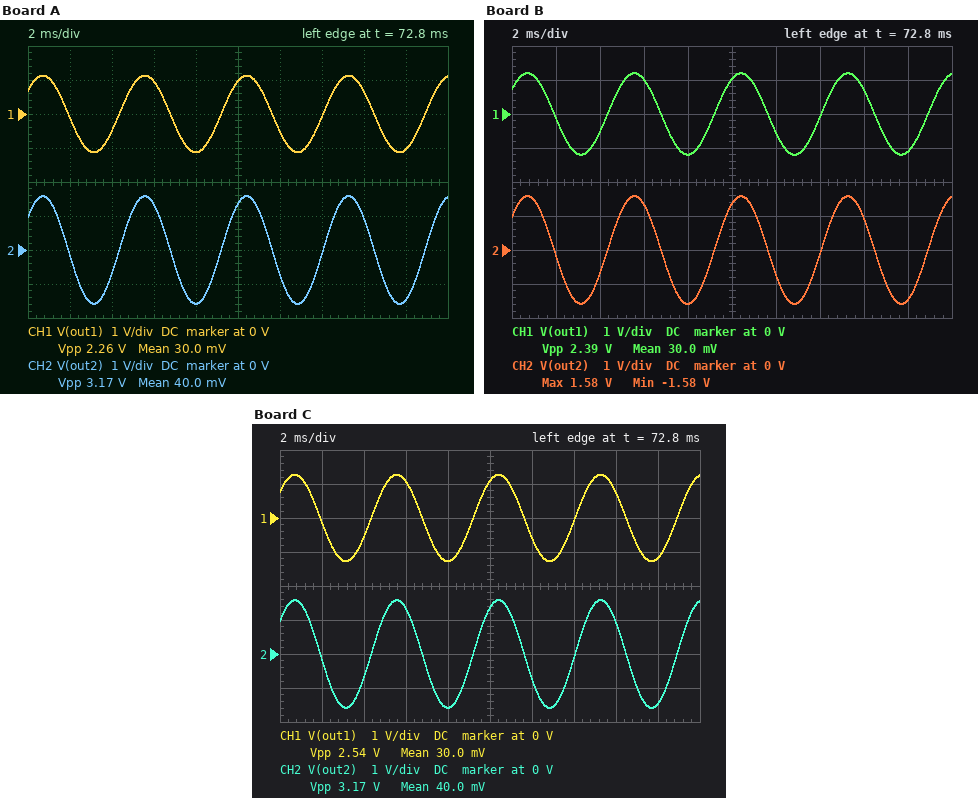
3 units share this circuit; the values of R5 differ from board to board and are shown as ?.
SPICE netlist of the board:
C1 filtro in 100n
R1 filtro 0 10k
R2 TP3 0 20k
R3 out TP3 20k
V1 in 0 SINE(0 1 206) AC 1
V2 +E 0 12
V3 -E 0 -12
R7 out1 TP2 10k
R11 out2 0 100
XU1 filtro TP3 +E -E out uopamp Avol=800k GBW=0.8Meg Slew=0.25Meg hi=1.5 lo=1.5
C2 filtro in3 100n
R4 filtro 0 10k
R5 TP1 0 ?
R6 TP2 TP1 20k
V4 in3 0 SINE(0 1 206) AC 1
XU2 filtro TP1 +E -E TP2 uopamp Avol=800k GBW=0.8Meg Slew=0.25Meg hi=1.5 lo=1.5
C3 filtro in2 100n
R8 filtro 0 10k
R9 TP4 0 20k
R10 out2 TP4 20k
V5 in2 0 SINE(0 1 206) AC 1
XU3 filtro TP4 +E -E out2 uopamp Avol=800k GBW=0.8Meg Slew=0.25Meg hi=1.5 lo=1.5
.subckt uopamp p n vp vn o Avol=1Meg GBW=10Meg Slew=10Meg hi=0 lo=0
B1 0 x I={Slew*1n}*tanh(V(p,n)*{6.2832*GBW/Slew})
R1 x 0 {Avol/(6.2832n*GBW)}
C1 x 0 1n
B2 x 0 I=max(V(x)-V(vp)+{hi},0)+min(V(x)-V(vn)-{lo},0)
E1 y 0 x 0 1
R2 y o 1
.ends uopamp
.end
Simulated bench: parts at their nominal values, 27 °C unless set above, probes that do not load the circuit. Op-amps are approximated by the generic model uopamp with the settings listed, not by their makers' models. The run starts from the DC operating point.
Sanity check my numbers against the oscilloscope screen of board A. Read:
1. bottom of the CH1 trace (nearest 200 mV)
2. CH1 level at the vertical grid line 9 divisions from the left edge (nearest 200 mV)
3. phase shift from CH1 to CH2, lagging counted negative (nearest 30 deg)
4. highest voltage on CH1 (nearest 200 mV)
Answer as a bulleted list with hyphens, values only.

- -1.2 V
- -1.0 V
- 0 deg
- 1.2 V
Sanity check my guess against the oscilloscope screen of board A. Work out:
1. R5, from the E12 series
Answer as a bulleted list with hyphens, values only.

- 47 kΩ
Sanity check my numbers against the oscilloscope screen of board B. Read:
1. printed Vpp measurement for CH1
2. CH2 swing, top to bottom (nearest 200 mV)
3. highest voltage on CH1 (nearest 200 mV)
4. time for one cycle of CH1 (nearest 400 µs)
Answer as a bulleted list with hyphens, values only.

- 2.39 V
- 3.2 V
- 1.2 V
- 4.8 ms
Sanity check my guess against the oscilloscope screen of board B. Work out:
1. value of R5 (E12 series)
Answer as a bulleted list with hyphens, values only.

- 39 kΩ
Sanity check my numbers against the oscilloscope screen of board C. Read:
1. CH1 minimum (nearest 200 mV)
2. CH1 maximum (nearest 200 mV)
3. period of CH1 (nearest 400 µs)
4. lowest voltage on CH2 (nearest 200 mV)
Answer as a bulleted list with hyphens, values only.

- -1.2 V
- 1.2 V
- 4.8 ms
- -1.6 V
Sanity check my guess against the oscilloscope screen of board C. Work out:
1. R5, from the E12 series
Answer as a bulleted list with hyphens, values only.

- 33 kΩ
